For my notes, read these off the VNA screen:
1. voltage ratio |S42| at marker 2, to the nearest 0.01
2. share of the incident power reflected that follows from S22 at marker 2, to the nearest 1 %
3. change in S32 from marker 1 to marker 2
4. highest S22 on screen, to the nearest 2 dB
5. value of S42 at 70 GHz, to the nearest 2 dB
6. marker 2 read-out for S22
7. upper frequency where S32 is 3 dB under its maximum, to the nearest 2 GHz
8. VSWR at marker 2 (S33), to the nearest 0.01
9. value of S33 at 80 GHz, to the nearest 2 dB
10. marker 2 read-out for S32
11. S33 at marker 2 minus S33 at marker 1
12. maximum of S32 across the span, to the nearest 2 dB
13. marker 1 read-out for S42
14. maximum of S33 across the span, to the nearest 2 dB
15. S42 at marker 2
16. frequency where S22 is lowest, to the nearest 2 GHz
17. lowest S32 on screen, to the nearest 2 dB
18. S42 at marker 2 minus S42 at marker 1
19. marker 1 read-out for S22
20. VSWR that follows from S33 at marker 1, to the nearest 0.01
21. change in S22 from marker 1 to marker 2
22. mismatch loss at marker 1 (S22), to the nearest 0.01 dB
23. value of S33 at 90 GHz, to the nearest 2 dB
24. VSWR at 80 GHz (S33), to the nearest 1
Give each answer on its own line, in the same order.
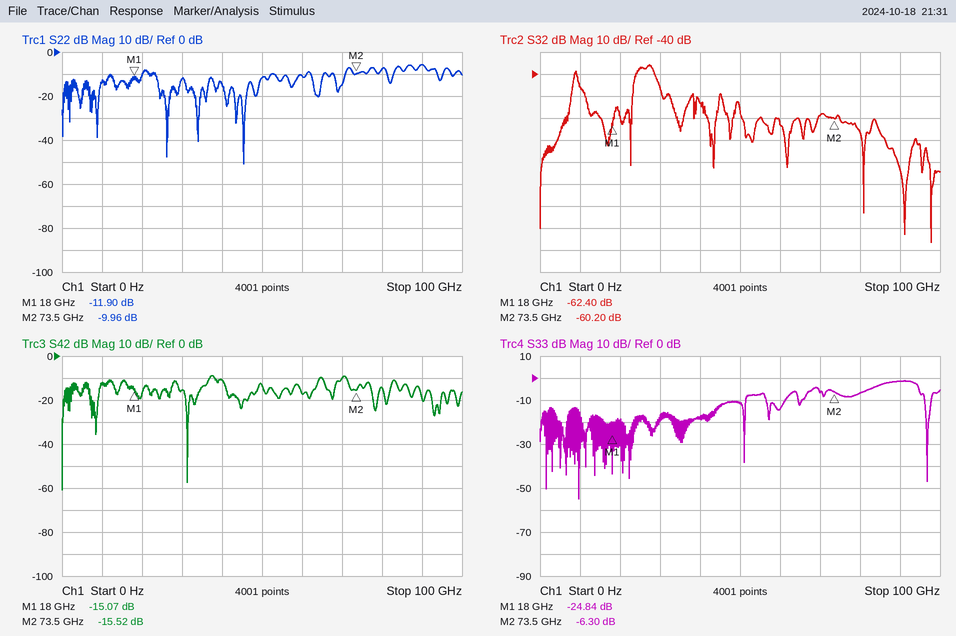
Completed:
0.17
10 %
2.20 dB
-6 dB
-10 dB
-9.96 dB
28 GHz
2.88
-6 dB
-60.20 dB
18.54 dB
-36 dB
-15.07 dB
-2 dB
-15.52 dB
46 GHz
-116 dB
-0.45 dB
-11.90 dB
1.12
1.94 dB
0.29 dB
-2 dB
3
